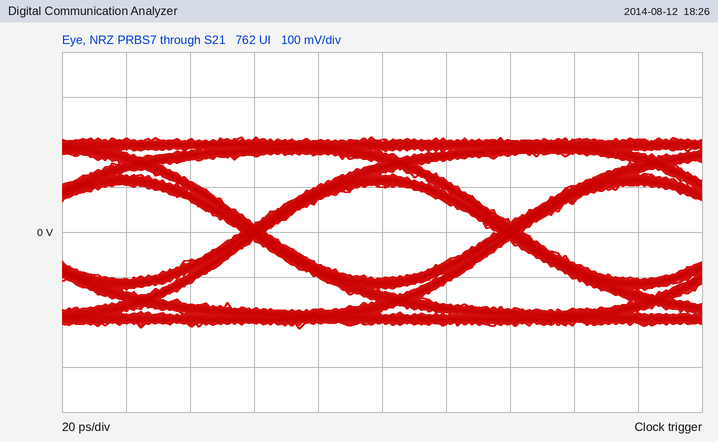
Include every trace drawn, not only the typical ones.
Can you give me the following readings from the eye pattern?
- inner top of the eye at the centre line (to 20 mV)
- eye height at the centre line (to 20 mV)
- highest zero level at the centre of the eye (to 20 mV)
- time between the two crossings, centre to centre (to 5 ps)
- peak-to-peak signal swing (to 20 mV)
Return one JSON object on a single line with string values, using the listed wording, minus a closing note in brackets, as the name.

{"inner top of the eye at the centre line": "100 mV", "eye height at the centre line": "200 mV", "highest zero level at the centre of the eye": "-100 mV", "time between the two crossings, centre to centre": "80 ps", "peak-to-peak signal swing": "420 mV"}
